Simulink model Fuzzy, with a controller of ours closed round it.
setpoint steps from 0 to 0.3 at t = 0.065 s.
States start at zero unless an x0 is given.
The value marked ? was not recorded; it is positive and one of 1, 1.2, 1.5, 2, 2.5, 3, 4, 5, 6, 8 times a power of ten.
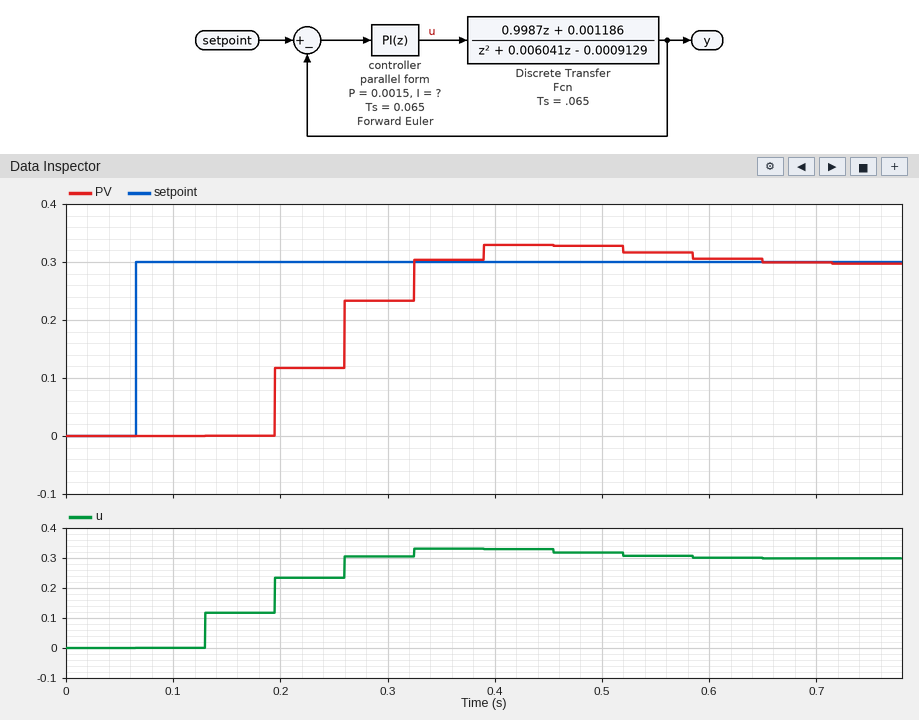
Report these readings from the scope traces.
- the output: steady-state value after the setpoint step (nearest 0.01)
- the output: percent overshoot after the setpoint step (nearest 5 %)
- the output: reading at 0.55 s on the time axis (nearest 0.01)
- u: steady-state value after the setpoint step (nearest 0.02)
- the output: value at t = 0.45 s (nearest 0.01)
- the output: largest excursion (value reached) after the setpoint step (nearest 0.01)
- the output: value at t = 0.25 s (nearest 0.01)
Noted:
0.30
10 %
0.32
0.30
0.33
0.33
0.12
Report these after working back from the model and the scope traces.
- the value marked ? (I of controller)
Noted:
6
